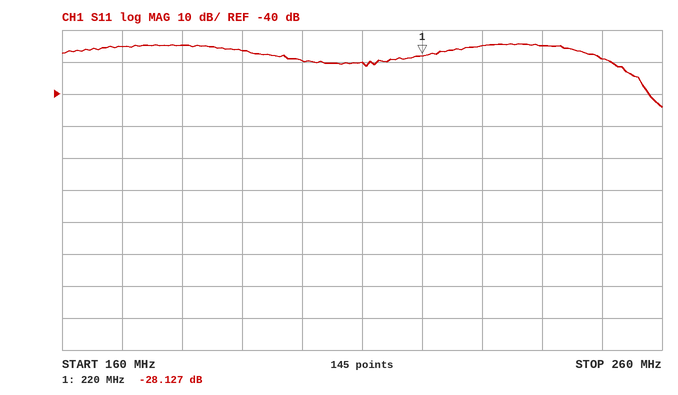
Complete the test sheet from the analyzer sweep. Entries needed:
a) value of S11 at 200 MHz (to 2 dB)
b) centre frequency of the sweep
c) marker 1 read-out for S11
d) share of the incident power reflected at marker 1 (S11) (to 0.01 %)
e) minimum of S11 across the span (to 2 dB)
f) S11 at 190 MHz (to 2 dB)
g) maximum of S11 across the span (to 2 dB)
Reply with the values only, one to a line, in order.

-30 dB
210 MHz
-28.127 dB
0.15 %
-44 dB
-26 dB
-24 dB
